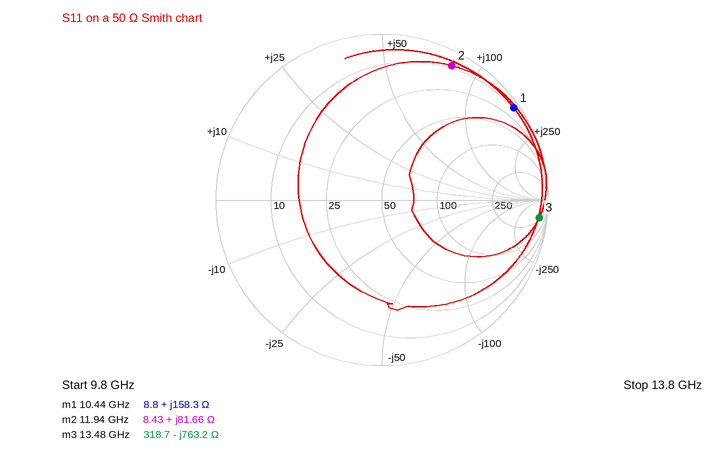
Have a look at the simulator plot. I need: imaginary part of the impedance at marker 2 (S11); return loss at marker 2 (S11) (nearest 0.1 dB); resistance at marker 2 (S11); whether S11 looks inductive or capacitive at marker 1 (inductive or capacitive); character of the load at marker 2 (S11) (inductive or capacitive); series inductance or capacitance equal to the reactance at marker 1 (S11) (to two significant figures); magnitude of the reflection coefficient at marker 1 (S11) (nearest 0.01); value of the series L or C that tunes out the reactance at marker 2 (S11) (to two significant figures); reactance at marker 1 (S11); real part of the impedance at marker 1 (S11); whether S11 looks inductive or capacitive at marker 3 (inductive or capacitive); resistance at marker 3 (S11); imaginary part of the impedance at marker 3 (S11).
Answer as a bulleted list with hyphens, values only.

- +81.66 Ω
- 0.8 dB
- 8.43 Ω
- inductive
- inductive
- 2.4 nH
- 0.97
- 160 fF
- +158.3 Ω
- 8.8 Ω
- capacitive
- 318.7 Ω
- -763.2 Ω
